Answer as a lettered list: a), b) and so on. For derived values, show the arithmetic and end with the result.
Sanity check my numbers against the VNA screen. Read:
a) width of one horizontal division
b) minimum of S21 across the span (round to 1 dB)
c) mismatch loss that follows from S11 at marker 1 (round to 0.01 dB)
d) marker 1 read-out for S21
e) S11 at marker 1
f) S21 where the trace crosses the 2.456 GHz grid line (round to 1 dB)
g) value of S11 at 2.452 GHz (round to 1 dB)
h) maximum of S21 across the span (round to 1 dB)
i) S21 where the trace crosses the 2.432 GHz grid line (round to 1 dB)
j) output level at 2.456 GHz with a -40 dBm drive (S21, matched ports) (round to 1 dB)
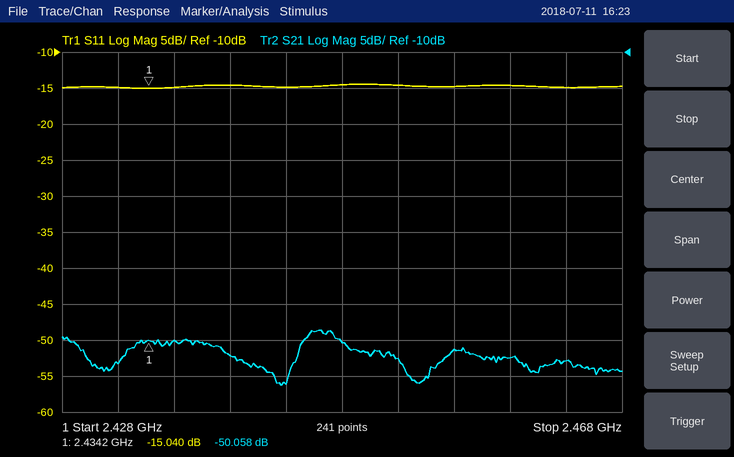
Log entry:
a) 4 MHz
b) -56 dB
c) −10 log10(1 − 10^(-15.04/10)) ≈ 0.14 dB
d) -50.058 dB
e) -15.040 dB
f) -51 dB
g) -15 dB
h) -49 dB
i) -53 dB
j) -40 dBm + (-51 dB) = -91 dBm
